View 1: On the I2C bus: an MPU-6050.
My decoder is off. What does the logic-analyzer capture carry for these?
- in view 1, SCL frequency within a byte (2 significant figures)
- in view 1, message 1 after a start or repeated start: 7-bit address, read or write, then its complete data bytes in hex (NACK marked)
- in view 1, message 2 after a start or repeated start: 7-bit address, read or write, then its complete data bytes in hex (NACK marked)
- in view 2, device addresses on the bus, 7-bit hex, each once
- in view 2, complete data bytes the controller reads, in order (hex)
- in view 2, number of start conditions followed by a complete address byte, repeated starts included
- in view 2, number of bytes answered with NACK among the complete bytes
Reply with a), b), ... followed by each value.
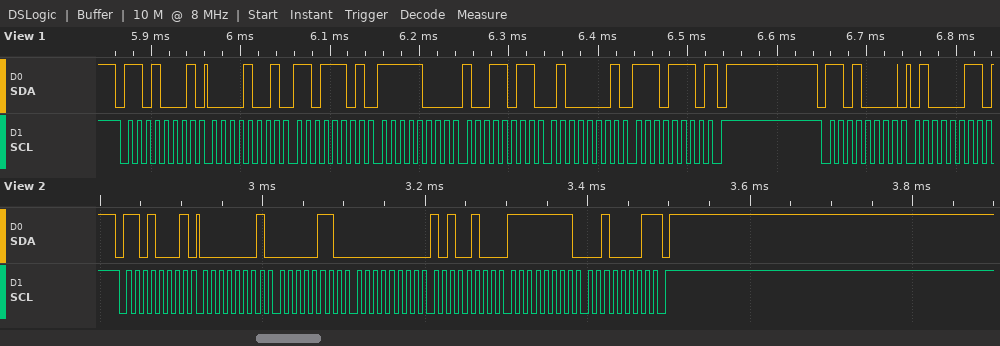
a) 100 kHz
b) 0x68 read: 09 DD F8 9B 41 EE NACK
c) 0x68 write: 43
d) 0x68
e) 01 06 00 A4 FF 21
f) 1
g) 1
